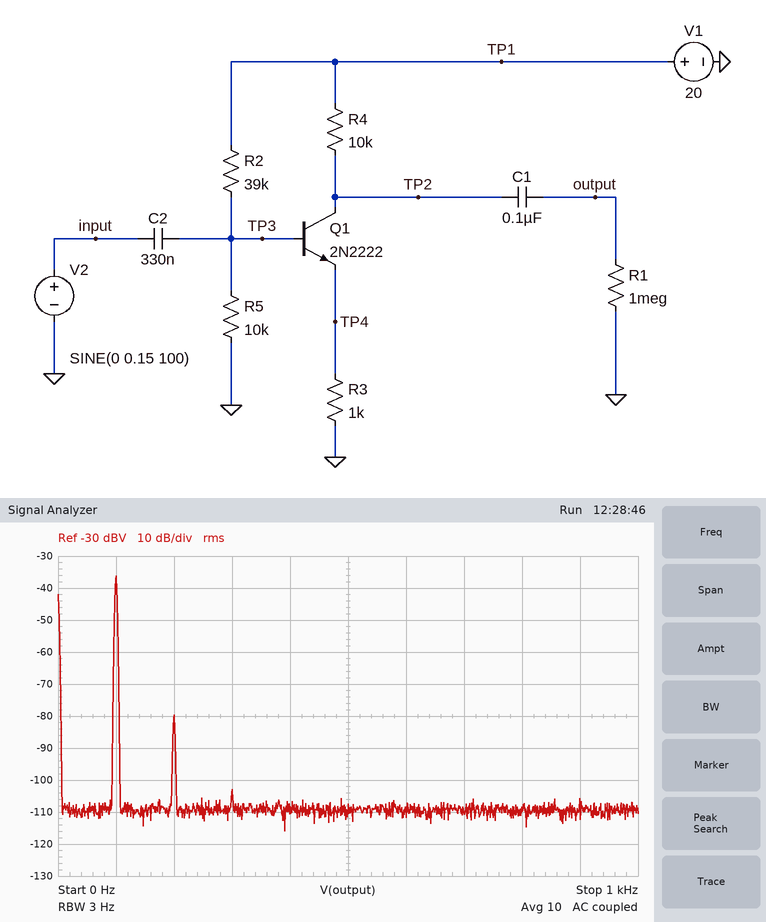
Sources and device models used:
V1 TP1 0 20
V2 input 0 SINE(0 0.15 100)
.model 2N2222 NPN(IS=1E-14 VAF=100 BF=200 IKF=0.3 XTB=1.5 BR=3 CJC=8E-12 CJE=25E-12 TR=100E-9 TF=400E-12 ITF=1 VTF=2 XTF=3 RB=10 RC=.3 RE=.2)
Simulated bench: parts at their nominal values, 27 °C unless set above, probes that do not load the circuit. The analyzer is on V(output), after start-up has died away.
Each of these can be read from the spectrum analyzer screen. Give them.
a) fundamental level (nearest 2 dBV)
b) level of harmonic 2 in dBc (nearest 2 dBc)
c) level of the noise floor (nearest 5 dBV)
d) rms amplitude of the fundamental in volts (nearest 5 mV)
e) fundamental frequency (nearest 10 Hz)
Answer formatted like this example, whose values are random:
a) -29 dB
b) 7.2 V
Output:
a) -36 dBV
b) -44 dBc
c) -110 dBV
d) 15 mV
e) 100 Hz
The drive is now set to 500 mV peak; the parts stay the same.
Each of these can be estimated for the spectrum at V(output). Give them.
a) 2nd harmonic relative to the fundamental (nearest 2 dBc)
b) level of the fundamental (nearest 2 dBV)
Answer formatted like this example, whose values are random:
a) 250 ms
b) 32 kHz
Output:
a) -32 dBc
b) -26 dBV
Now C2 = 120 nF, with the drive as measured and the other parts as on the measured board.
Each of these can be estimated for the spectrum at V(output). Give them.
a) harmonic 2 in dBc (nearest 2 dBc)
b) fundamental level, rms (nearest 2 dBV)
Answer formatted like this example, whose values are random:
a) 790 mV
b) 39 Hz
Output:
a) -52 dBc
b) -44 dBV
